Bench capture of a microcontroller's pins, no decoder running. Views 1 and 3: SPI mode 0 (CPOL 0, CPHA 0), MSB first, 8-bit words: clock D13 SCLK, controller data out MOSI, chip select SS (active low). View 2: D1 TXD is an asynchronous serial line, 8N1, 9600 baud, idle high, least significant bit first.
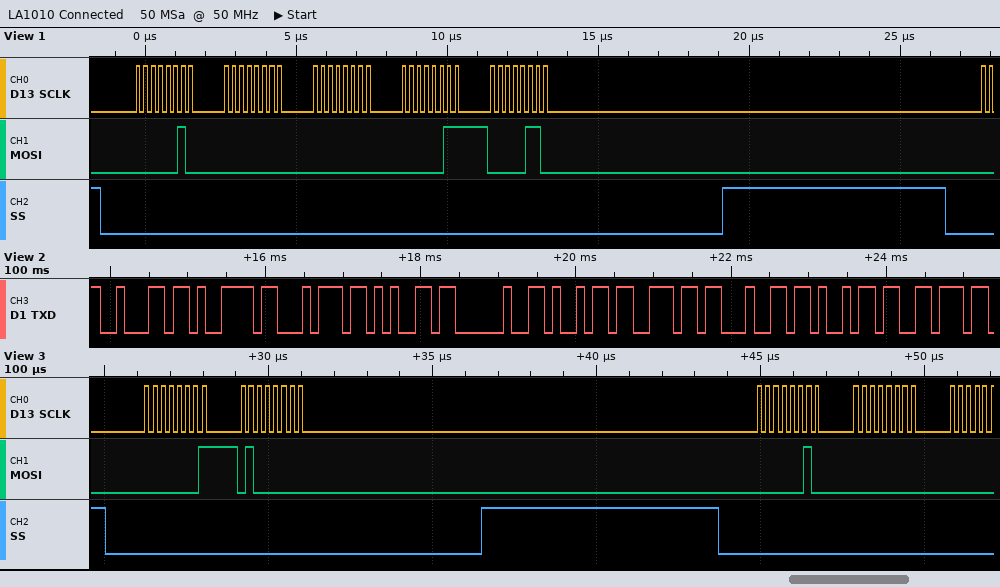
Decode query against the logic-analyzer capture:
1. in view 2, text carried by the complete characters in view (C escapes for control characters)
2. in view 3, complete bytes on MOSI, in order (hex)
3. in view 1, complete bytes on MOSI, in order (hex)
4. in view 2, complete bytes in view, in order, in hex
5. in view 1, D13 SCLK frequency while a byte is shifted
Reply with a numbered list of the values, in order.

1. "byte indiv"
2. 0x01 0x40 0x02 0x00
3. 02 00 00 03 06
4. 62 79 74 65 20 69 6E 64 69 76
5. 4 MHz
